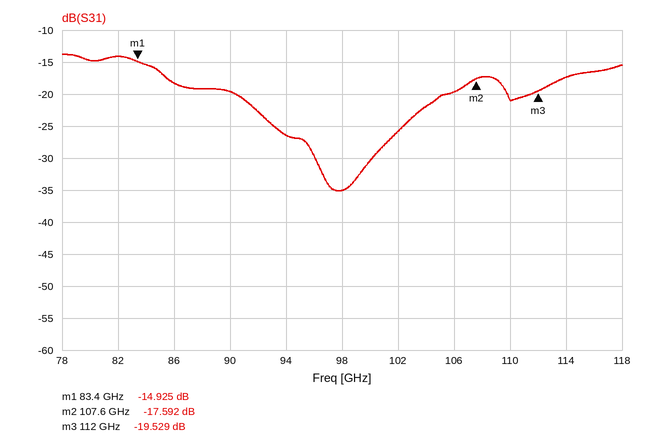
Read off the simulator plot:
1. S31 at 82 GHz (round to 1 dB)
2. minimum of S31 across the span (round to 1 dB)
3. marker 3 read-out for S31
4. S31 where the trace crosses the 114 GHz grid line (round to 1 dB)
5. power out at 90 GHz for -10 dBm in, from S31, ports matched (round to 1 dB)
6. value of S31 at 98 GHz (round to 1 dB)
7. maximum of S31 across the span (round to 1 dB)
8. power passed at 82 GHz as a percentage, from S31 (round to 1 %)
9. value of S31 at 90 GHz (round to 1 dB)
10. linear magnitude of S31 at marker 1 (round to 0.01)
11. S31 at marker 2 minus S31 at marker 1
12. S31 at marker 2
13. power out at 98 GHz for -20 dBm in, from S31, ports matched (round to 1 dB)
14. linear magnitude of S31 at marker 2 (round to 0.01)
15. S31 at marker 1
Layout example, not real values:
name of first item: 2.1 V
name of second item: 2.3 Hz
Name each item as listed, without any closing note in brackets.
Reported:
S31 at 82 GHz: -14 dB
minimum of S31 across the span: -35 dB
marker 3 read-out for S31: -19.529 dB
S31 where the trace crosses the 114 GHz grid line: -17 dB
power out at 90 GHz for -10 dBm in, from S31, ports matched: -30 dBm
value of S31 at 98 GHz: -35 dB
maximum of S31 across the span: -14 dB
power passed at 82 GHz as a percentage, from S31: 4 %
value of S31 at 90 GHz: -20 dB
linear magnitude of S31 at marker 1: 0.18
S31 at marker 2 minus S31 at marker 1: -2.667 dB
S31 at marker 2: -17.592 dB
power out at 98 GHz for -20 dBm in, from S31, ports matched: -55 dBm
linear magnitude of S31 at marker 2: 0.13
S31 at marker 1: -14.925 dB
